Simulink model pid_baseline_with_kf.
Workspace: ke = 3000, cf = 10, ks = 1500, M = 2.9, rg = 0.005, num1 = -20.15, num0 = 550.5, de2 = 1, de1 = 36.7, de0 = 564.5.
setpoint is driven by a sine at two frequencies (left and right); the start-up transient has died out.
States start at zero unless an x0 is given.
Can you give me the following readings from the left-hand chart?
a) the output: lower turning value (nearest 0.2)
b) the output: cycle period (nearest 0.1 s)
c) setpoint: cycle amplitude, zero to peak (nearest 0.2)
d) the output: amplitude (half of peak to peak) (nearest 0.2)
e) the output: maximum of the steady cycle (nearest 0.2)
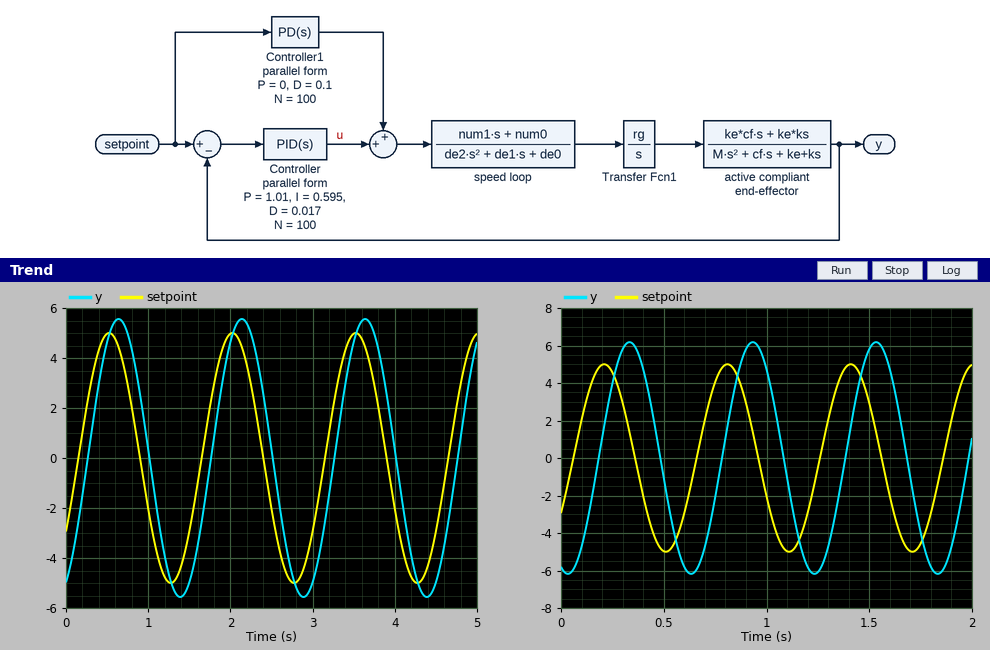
-5.6
1.5 s
5.0
5.6
5.6
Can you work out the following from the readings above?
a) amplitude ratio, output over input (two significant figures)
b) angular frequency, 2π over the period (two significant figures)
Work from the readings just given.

1.1
4.2 rad/s
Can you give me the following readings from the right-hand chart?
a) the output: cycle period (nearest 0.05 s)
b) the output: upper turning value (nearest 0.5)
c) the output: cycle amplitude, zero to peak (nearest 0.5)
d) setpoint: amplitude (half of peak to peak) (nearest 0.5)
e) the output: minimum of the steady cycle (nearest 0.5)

0.60 s
6.0
6.0
5.0
-6.0
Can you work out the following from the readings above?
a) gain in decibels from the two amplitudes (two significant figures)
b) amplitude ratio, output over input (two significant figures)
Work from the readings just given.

1.6 dB
1.2
